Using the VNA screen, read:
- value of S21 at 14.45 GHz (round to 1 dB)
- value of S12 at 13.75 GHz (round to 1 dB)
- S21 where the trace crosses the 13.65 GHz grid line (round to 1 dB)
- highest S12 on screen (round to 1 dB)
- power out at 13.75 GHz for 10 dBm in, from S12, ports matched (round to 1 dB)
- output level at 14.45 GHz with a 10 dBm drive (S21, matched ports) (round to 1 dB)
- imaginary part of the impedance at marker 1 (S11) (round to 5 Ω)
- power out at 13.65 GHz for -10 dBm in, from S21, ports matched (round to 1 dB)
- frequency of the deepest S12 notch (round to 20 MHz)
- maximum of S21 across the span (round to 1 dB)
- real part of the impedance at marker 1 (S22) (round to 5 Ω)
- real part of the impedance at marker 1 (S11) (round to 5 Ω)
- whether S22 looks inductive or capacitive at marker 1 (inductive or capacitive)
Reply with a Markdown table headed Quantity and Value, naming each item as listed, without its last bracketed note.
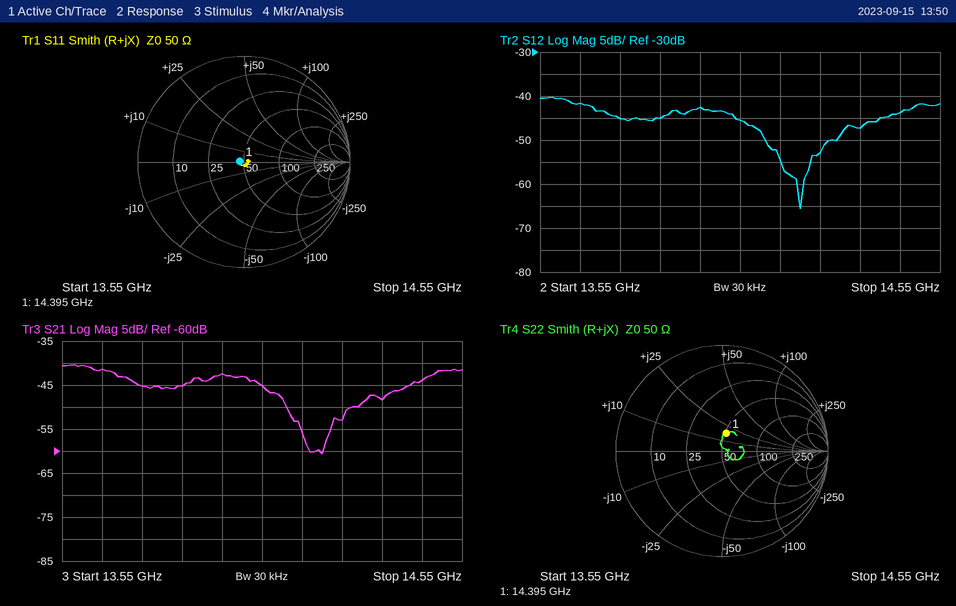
| Quantity | Value |
|---|---|
| value of S21 at 14.45 GHz | -44 dB |
| value of S12 at 13.75 GHz | -45 dB |
| S21 where the trace crosses the 13.65 GHz grid line | -41 dB |
| highest S12 on screen | -40 dB |
| power out at 13.75 GHz for 10 dBm in, from S12, ports matched | -35 dBm |
| output level at 14.45 GHz with a 10 dBm drive (S21, matched ports) | -34 dBm |
| imaginary part of the impedance at marker 1 (S11) | 0 Ω |
| power out at 13.65 GHz for -10 dBm in, from S21, ports matched | -51 dBm |
| frequency of the deepest S12 notch | 14.20 GHz |
| maximum of S21 across the span | -40 dB |
| real part of the impedance at marker 1 (S22) | 50 Ω |
| real part of the impedance at marker 1 (S11) | 45 Ω |
| whether S22 looks inductive or capacitive at marker 1 | inductive |
